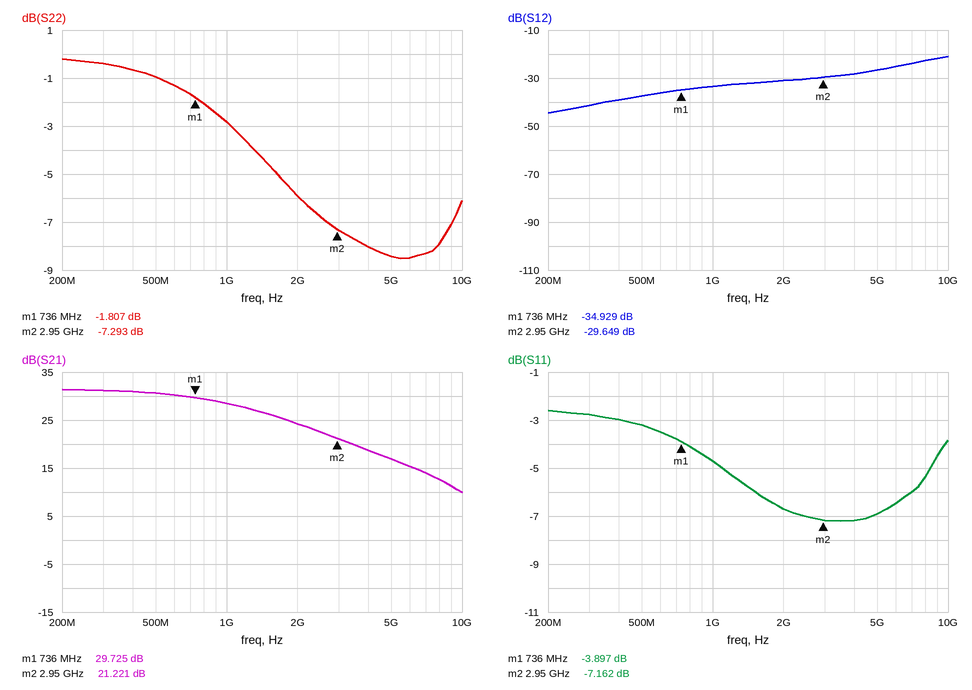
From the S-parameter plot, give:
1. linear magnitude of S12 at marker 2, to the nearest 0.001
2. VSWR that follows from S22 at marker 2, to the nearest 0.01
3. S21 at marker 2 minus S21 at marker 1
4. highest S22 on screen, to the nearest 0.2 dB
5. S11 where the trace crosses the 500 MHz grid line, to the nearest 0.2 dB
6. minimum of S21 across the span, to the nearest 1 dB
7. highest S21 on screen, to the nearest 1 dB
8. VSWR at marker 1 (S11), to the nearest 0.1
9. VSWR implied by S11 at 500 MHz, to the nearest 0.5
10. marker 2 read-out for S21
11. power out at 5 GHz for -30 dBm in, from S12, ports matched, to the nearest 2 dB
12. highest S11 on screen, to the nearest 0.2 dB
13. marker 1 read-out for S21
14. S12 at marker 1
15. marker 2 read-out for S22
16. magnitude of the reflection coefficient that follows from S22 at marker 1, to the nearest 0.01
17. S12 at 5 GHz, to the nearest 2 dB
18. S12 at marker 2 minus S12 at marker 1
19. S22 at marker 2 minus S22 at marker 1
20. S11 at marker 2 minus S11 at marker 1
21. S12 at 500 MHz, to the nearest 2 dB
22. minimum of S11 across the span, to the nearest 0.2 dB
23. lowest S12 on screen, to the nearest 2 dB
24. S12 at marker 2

0.033
2.52
-8.504 dB
-0.2 dB
-3.2 dB
10 dB
31 dB
4.5
5.5
21.221 dB
-56 dBm
-2.6 dB
29.725 dB
-34.929 dB
-7.293 dB
0.81
-26 dB
5.280 dB
-5.486 dB
-3.265 dB
-38 dB
-7.2 dB
-44 dB
-29.649 dB
